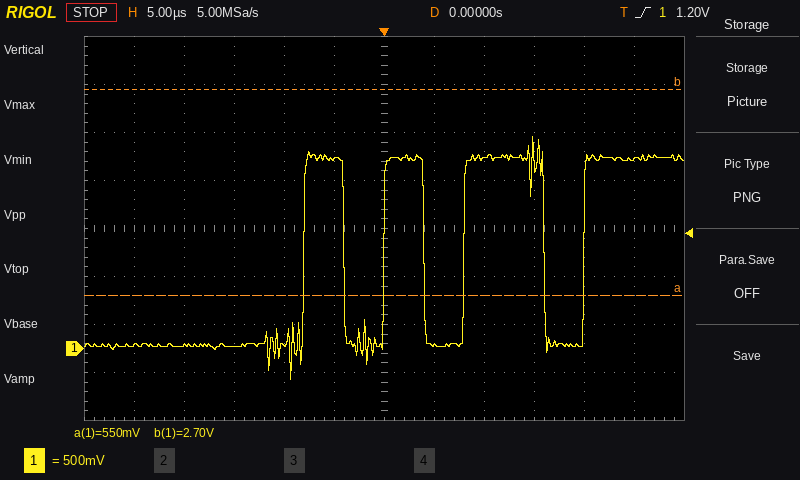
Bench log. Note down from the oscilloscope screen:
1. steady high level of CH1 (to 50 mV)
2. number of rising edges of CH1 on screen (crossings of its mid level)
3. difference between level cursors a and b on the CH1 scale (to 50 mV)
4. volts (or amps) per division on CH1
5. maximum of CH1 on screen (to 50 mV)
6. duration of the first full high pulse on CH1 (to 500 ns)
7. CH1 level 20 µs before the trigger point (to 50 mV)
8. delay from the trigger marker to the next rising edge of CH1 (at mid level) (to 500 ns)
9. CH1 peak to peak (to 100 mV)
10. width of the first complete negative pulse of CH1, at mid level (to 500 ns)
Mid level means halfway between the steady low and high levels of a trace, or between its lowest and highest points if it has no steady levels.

2.00 V
4
2.15 V
500 mV
2.20 V
4.0 µs
50 mV
8.0 µs
2.50 V
4.0 µs
